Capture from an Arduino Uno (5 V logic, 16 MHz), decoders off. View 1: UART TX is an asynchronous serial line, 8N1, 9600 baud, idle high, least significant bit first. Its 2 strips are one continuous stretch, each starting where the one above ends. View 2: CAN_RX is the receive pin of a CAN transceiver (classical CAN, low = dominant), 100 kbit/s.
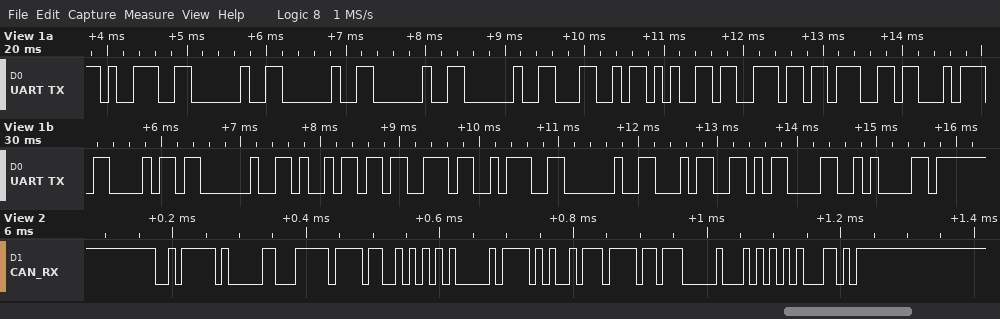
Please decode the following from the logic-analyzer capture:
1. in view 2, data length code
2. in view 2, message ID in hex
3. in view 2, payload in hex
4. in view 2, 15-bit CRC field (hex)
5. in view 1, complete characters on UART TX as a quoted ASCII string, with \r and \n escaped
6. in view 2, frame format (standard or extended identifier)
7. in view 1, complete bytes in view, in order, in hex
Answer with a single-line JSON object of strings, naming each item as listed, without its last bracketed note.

{"in view 2, data length code": "8", "in view 2, message ID in hex": "0x2FC", "in view 2, payload in hex": "FF B2 AA 07 A9 77 B7 00", "in view 2, 15-bit CRC field": "0x5546", "in view 1, complete characters on UART TX as a quoted ASCII string, with \\r and \\n escaped": "\"9    Length is: 4\\r\\n\"", "in view 2, frame format": "standard", "in view 1, complete bytes in view, in order, in hex": "39 20 20 20 20 4C 65 6E 67 74 68 20 69 73 3A 20 34 0D 0A"}
